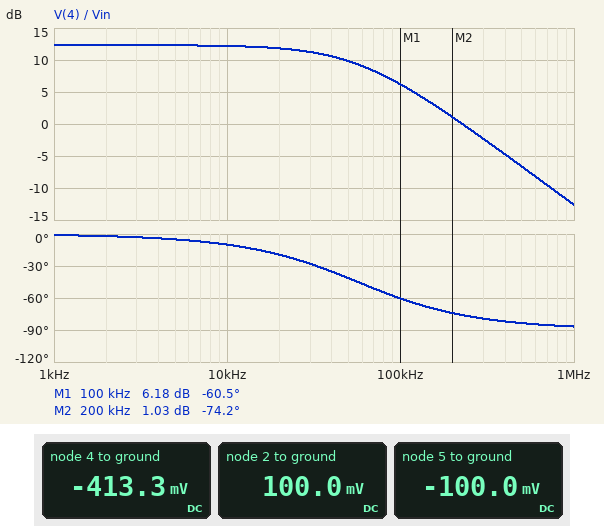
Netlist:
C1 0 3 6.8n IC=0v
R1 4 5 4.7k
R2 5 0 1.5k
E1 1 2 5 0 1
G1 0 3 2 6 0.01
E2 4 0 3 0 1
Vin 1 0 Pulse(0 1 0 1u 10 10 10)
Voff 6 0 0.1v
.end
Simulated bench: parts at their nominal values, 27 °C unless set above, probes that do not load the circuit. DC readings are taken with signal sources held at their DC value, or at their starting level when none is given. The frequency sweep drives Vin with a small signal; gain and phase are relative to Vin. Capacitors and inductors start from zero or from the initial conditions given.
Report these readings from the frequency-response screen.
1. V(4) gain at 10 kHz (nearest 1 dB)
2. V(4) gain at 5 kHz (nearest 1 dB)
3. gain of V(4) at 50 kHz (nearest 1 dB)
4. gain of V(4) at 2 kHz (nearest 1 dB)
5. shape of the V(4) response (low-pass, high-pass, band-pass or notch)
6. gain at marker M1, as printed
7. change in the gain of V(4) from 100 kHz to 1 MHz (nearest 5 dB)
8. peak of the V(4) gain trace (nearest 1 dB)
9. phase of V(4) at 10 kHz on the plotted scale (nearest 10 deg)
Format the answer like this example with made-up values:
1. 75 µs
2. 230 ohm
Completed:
1. 12 dB
2. 12 dB
3. 10 dB
4. 12 dB
5. low-pass
6. 6.18 dB
7. -20 dB
8. 12 dB
9. -10 deg
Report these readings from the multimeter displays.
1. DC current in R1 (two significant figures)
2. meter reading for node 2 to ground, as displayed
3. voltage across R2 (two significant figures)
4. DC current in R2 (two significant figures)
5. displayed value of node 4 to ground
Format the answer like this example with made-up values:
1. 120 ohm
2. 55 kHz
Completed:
1. 67 µA
2. 100.0 mV
3. 100 mV
4. 67 µA
5. -413.3 mV
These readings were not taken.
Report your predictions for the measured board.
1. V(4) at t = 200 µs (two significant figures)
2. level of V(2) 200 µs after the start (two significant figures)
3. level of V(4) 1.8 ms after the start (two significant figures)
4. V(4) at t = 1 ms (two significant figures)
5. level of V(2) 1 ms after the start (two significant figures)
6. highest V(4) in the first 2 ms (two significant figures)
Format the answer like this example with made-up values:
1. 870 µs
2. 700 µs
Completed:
1. 3.7 V
2. 100 mV
3. 3.7 V
4. 3.7 V
5. 100 mV
6. 3.7 V
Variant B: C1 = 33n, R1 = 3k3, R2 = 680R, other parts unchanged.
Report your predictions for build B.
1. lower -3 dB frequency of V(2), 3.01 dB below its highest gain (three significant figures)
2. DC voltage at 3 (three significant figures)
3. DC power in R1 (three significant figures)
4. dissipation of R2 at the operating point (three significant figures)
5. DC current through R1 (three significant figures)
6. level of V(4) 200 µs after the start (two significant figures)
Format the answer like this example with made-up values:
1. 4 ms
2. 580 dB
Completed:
1. 8.24 kHz
2. -585 mV
3. 71.4 µW
4. 14.7 µW
5. 147 µA
6. 5.3 V
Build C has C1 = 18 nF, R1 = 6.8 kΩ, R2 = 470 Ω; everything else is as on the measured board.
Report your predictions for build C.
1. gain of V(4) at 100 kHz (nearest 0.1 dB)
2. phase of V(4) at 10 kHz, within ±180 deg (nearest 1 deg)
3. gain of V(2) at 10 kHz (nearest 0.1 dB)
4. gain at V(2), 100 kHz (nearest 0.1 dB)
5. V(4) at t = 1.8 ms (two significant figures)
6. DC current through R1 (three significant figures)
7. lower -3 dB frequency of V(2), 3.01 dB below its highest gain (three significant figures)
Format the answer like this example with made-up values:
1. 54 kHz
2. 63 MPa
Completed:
1. -1.1 dB
2. -60 deg
3. -1.2 dB
4. 0 dB
5. 14 V
6. 213 µA
7. 5.72 kHz
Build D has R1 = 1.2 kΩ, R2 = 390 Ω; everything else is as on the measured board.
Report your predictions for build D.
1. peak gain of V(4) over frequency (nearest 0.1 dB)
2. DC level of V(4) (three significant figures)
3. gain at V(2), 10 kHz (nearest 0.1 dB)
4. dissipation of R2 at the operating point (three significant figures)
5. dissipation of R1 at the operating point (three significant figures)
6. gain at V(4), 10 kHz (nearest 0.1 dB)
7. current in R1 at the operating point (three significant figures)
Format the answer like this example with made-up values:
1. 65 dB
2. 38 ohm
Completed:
1. 12.2 dB
2. -408 mV
3. -15.3 dB
4. 25.6 µW
5. 78.9 µW
6. 12.1 dB
7. 256 µA
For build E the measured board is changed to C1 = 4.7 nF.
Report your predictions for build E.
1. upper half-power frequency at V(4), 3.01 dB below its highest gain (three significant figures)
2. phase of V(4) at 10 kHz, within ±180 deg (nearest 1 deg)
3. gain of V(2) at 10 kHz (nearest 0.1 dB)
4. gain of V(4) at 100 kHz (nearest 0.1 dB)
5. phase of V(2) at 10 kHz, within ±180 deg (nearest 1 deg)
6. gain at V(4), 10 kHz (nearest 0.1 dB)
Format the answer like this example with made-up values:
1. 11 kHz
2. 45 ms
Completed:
1. 81.9 kHz
2. -7 deg
3. -18.3 dB
4. 8.4 dB
5. 83 deg
6. 12.3 dB
